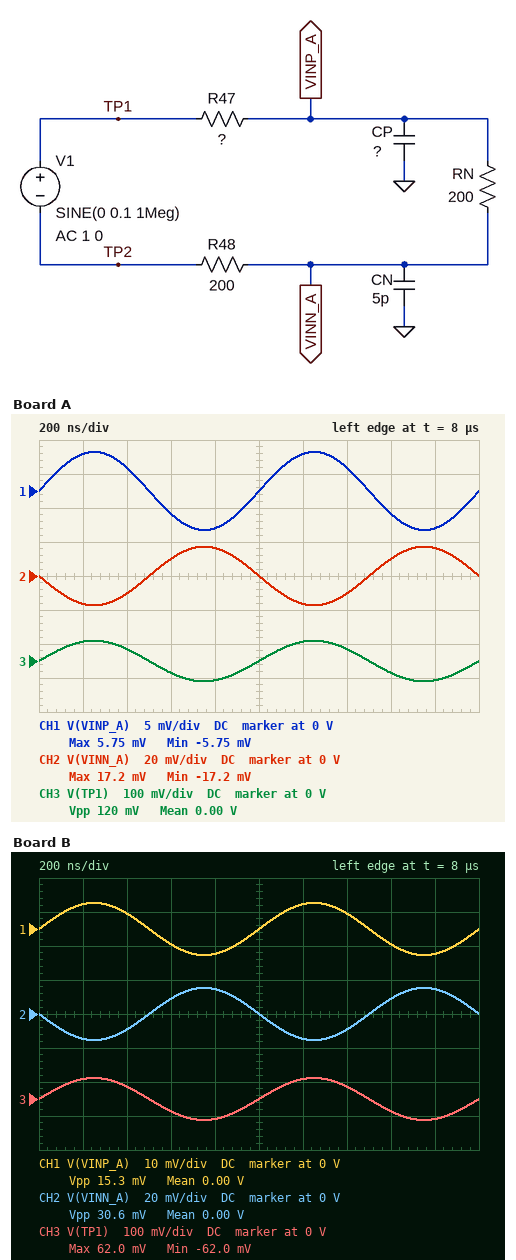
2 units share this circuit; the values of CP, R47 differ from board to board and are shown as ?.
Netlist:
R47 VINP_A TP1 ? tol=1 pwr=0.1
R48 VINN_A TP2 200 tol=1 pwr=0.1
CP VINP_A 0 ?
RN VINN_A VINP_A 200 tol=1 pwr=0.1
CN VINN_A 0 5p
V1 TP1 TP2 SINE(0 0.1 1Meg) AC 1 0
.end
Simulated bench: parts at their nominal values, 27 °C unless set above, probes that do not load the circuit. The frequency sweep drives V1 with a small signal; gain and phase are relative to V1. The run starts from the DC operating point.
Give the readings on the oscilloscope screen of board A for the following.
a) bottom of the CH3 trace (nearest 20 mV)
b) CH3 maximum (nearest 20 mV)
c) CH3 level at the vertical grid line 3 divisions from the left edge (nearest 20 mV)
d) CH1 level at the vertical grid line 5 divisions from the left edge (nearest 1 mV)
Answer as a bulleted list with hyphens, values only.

- -60 mV
- 60 mV
- -40 mV
- 0 V
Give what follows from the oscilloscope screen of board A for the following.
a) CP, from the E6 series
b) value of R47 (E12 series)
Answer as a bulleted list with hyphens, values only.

- 15 pF
- 470 Ω
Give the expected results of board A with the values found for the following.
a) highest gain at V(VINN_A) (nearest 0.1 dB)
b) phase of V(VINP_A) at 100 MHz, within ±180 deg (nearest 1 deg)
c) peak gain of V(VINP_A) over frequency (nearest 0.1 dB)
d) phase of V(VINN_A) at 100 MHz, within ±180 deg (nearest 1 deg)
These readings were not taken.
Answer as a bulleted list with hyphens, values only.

- -15.3 dB
- -20 deg
- -24.8 dB
- 160 deg
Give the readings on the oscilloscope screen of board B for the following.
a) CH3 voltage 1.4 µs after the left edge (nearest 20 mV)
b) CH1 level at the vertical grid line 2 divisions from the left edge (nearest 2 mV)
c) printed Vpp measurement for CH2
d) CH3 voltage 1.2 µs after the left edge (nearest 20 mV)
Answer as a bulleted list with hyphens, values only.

- 40 mV
- 4 mV
- 30.6 mV
- 60 mV
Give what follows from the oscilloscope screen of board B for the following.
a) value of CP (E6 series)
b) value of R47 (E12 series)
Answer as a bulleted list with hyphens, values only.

- 10 pF
- 470 Ω
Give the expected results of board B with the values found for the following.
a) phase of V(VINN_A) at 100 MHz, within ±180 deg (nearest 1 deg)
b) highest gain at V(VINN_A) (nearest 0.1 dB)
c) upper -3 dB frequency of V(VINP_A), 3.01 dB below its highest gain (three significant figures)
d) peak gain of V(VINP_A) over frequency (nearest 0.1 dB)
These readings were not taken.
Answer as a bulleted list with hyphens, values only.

- 162 deg
- -16.3 dB
- 310 MHz
- -22.3 dB
